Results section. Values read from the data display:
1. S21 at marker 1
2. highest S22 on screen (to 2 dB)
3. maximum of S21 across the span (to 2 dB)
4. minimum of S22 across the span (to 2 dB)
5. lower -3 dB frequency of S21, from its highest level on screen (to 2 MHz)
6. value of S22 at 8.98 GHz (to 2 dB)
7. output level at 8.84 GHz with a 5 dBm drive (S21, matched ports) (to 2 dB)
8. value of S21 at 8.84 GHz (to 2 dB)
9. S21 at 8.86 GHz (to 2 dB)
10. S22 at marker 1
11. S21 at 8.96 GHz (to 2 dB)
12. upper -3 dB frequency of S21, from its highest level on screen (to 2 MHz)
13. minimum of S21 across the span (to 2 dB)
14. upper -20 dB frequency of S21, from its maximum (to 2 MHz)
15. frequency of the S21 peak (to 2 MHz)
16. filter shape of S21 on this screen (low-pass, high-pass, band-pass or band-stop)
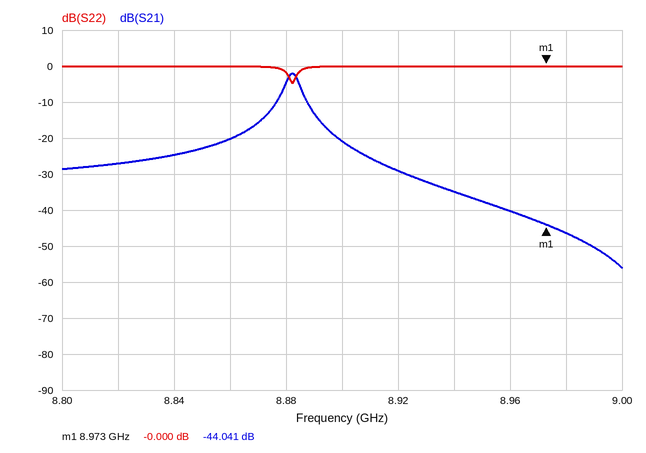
-44.041 dB
0 dB
-2 dB
-4 dB
8.880 GHz
0 dB
-20 dBm
-24 dB
-20 dB
-0.000 dB
-40 dB
8.884 GHz
-56 dB
8.902 GHz
8.882 GHz
band-pass
